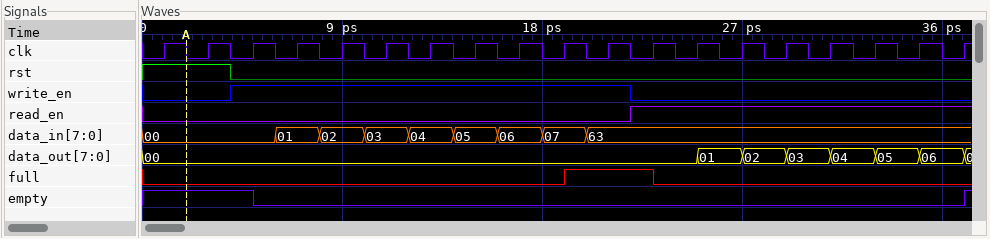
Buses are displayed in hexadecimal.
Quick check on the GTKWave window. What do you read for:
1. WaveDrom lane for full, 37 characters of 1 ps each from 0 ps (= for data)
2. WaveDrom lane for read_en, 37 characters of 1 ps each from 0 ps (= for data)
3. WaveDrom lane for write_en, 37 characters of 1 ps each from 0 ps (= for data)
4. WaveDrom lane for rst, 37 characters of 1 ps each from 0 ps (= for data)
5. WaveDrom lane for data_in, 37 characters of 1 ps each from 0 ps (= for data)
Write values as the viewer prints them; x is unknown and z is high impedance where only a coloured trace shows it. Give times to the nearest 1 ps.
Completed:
{name: 'full', wave: '0..................1...0.............'}
{name: 'read_en', wave: '0.....................1..............'}
{name: 'write_en', wave: '0...1.................0..............'}
{name: 'rst', wave: '1...0................................'}
{name: 'data_in', wave: '=.....=.=.=.=.=.=.=.=................', data: '00 01 02 03 04 05 06 07 63'}
